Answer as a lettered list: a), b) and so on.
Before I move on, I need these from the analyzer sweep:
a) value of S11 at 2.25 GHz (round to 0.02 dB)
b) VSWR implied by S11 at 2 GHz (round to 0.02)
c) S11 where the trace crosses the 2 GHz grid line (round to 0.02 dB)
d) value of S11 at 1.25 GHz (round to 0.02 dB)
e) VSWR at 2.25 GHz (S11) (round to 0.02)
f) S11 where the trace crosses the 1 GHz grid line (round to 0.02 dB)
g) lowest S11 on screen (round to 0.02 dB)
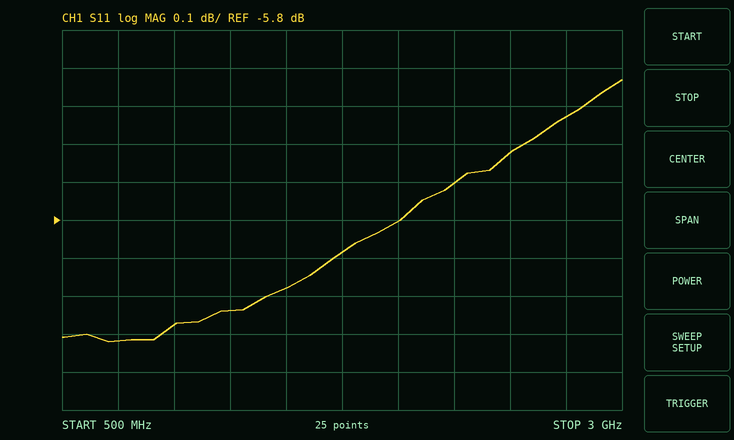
a) -5.70 dB
b) 3.10
c) -5.80 dB
d) -6.04 dB
e) 3.16
f) -6.08 dB
g) -6.12 dB
